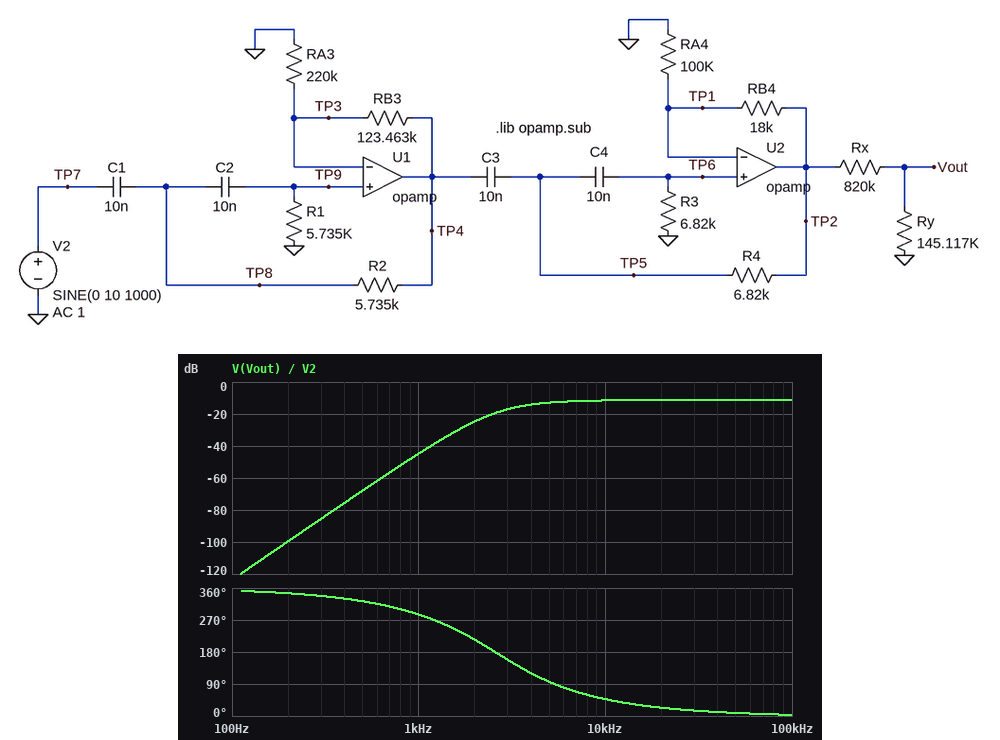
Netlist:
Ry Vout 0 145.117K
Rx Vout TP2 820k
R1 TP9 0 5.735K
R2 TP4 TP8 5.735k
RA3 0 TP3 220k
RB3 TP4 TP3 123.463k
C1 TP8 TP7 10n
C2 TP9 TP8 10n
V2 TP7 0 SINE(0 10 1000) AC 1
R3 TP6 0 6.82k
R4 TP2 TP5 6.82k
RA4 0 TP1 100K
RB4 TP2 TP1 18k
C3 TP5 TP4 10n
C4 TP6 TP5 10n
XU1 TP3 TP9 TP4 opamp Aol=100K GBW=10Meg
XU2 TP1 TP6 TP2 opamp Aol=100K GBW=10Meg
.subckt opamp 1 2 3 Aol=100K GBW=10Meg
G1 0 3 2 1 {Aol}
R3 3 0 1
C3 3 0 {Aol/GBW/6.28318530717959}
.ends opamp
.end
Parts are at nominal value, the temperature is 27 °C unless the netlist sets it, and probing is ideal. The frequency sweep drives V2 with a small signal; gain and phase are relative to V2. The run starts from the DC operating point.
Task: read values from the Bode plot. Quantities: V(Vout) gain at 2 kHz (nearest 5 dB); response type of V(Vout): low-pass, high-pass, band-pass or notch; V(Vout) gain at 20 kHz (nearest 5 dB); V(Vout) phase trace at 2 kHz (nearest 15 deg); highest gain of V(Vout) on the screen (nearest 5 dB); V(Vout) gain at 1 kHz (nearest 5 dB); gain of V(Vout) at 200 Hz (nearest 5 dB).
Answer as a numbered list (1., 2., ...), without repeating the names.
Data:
1. -25 dB
2. high-pass
3. -10 dB
4. 210 deg
5. -10 dB
6. -45 dB
7. -100 dB
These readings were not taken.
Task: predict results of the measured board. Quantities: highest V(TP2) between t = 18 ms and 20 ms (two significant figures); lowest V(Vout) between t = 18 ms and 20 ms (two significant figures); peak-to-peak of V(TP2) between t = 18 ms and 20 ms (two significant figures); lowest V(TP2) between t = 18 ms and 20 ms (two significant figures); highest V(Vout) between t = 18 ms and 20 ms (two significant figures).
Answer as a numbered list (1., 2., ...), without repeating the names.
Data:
1. 380 mV
2. -58 mV
3. 770 mV
4. -380 mV
5. 58 mV
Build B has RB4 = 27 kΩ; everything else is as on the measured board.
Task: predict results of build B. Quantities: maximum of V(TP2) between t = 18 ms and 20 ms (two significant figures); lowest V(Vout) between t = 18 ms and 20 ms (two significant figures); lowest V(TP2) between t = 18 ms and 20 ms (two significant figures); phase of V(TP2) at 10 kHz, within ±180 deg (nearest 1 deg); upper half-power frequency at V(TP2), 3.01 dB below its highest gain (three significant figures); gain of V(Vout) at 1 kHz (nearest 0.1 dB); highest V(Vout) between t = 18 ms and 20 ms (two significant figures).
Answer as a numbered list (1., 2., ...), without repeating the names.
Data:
1. 420 mV
2. -64 mV
3. -420 mV
4. 46 deg
5. 4.54 MHz
6. -43.9 dB
7. 64 mV
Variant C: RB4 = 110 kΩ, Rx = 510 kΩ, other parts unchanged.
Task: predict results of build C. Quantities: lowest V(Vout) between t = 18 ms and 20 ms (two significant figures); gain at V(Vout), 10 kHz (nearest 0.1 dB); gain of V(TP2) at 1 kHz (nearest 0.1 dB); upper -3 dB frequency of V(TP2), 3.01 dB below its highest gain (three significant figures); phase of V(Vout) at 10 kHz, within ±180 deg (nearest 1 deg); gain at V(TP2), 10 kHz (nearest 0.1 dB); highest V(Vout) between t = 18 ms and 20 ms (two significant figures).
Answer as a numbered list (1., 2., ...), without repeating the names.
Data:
1. -190 mV
2. -2.6 dB
3. -21.4 dB
4. 3.10 MHz
5. 36 deg
6. 10.5 dB
7. 190 mV
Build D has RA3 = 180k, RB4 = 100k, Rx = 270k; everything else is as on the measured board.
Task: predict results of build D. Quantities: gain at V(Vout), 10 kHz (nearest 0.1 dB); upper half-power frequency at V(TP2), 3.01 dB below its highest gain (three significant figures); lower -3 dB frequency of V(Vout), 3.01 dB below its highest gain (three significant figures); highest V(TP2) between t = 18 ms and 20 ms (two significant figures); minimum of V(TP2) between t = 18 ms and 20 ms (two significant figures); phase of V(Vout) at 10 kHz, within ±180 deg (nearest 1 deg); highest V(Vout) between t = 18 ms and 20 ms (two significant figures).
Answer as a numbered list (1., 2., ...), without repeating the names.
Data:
1. 1.7 dB
2. 2.93 MHz
3. 2.60 kHz
4. 880 mV
5. -880 mV
6. 35 deg
7. 310 mV
